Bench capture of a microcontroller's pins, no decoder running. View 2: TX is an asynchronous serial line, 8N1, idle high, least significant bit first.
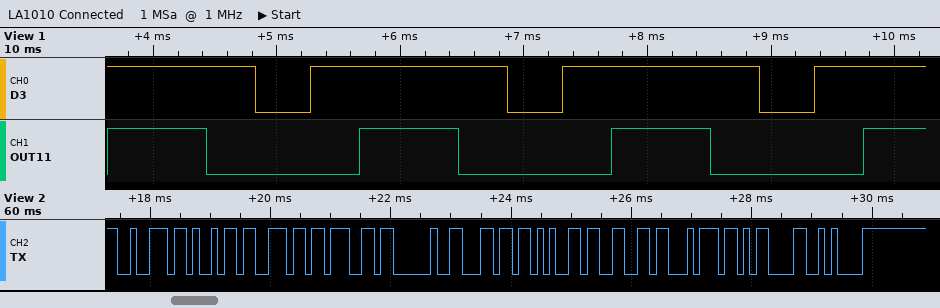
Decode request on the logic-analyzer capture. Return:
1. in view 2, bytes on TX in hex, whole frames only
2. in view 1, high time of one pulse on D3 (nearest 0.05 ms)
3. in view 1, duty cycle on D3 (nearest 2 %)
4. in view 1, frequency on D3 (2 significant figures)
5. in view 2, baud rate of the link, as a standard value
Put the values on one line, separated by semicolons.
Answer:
0x72 0x69 0x6E 0x67 0x20 0x6C 0x65 0x66 0x74 0x0D 0x0A; 1.60 ms; 78 %; 490 Hz; 9600 baud
